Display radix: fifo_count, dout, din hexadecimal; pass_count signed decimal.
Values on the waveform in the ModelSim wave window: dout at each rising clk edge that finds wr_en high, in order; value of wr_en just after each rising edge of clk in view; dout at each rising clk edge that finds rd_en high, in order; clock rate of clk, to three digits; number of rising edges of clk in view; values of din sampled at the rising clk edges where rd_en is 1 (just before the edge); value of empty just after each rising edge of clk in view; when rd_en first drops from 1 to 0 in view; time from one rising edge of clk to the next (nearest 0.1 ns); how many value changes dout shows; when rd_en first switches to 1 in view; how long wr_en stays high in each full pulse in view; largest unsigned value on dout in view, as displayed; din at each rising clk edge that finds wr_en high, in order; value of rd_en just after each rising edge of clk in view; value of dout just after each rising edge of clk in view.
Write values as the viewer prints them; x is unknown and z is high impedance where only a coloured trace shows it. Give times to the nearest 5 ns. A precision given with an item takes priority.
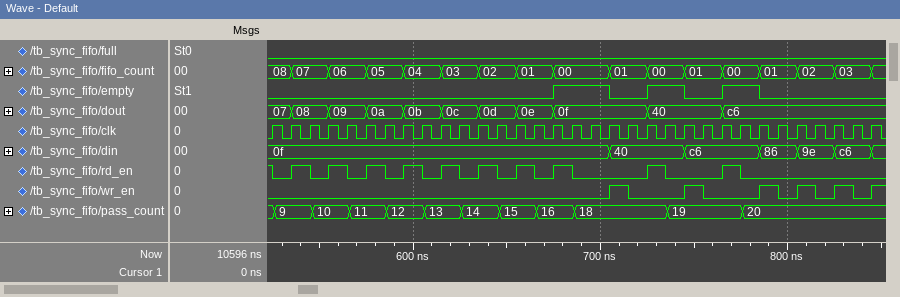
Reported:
0f, 40, c6, c6, c6
0 0 0 0 0 0 0 0 0 0 0 0 0 0 0 0 0 0 1 0 0 0 1 0 0 0 1 0 1 0 1 0 1
07, 08, 09, 0a, 0b, 0c, 0d, 0e, 0f, 40, c6
100 MHz
33
0f, 0f, 0f, 0f, 0f, 0f, 0f, 0f, 0f, 40, c6
0 0 0 0 0 0 0 0 0 0 0 0 0 0 0 1 1 1 0 0 1 1 0 0 1 1 0 0 0 0 0 0 0
525 ns
10 ns
10
535 ns
10 ns, 10 ns, 10 ns, 10 ns, 10 ns
c6
40, c6, 86, 9e, c6
0 1 0 1 0 1 0 1 0 1 0 1 0 1 0 1 0 0 0 0 1 0 0 0 1 0 0 0 0 0 0 0 0
07, 08, 08, 09, 09, 0a, 0a, 0b, 0b, 0c, 0c, 0d, 0d, 0e, 0e, 0f, 0f, 0f, 0f, 0f, 40, 40, 40, 40, c6, c6, c6, c6, c6, c6, c6, c6, c6
